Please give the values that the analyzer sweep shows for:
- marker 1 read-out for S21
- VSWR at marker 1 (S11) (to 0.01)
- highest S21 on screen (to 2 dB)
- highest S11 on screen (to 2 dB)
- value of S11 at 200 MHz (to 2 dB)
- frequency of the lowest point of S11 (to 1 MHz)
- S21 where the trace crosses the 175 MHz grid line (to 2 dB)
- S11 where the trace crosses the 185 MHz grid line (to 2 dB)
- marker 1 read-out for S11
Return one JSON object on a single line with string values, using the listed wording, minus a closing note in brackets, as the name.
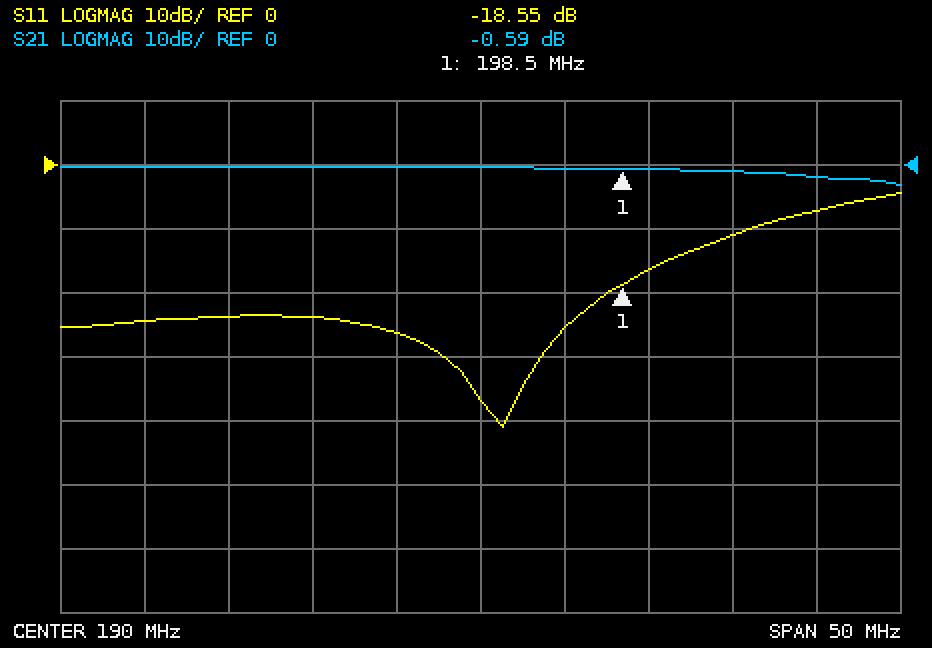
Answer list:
{"marker 1 read-out for S21": "-0.59 dB", "VSWR at marker 1 (S11)": "1.27", "highest S21 on screen": "0 dB", "highest S11 on screen": "-4 dB", "value of S11 at 200 MHz": "-16 dB", "frequency of the lowest point of S11": "191 MHz", "S21 where the trace crosses the 175 MHz grid line": "0 dB", "S11 where the trace crosses the 185 MHz grid line": "-26 dB", "marker 1 read-out for S11": "-18.55 dB"}
